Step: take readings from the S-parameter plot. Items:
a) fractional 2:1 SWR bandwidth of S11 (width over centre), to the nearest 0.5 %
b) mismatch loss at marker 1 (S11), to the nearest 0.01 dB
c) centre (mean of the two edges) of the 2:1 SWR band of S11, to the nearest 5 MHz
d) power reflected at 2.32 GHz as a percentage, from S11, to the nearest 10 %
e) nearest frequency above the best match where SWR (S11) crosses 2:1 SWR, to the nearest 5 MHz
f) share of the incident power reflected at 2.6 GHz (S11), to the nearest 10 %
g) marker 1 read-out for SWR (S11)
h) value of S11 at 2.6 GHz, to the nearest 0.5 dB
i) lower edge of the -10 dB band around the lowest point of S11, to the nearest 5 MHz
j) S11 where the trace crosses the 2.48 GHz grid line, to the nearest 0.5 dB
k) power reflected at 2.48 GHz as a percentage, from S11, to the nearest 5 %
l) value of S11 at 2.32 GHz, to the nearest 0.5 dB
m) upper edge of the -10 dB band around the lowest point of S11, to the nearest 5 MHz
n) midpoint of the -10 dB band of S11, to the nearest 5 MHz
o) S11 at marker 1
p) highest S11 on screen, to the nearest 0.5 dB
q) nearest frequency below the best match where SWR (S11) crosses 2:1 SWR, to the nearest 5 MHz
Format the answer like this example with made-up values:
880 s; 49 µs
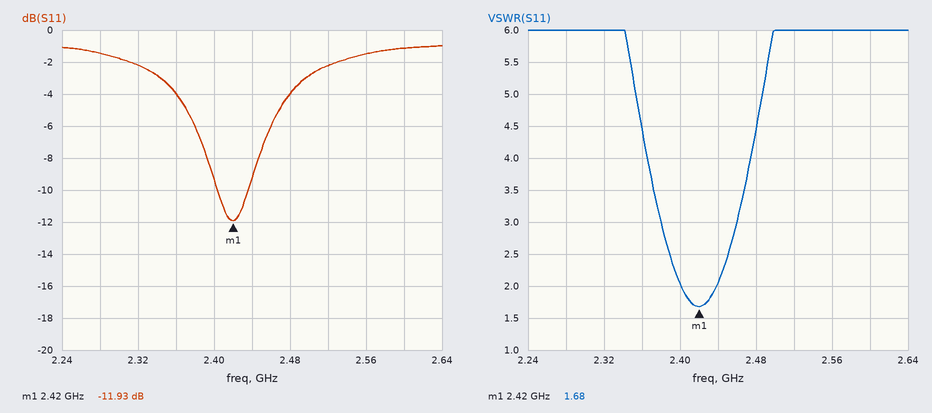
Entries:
1.5 %; 0.29 dB; 2.420 GHz; 60 %; 2.440 GHz; 80 %; 1.68; -1.0 dB; 2.405 GHz; -4.0 dB; 40 %; -2.0 dB; 2.435 GHz; 2.420 GHz; -11.93 dB; -1.0 dB; 2.400 GHz
